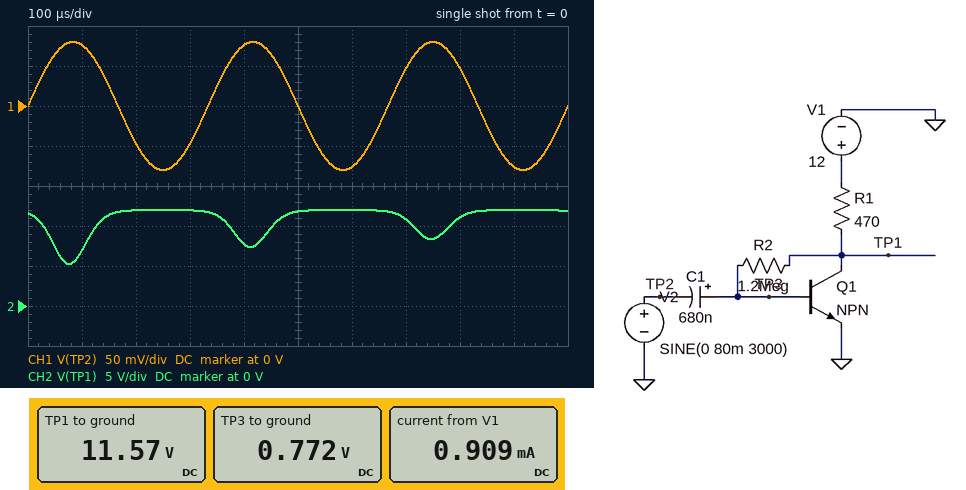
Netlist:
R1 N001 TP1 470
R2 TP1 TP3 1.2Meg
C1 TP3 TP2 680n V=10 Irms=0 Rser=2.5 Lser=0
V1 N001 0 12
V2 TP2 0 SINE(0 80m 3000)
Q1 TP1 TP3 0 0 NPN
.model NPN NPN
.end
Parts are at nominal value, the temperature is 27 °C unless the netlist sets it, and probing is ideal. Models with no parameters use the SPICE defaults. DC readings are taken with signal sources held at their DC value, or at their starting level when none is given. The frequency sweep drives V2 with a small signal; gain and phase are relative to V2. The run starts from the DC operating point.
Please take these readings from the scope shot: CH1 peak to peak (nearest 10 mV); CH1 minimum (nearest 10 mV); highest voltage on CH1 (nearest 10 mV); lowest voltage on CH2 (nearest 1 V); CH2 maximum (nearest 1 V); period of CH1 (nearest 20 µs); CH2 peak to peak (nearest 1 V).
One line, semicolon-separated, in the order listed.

160 mV; -80 mV; 80 mV; 5 V; 12 V; 340 µs; 7 V
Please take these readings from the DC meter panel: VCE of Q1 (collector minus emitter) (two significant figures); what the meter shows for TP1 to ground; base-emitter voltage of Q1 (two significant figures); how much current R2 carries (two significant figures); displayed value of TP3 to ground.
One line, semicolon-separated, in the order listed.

12 V; 11.57 V; 770 mV; 9.0 µA; 0.772 V
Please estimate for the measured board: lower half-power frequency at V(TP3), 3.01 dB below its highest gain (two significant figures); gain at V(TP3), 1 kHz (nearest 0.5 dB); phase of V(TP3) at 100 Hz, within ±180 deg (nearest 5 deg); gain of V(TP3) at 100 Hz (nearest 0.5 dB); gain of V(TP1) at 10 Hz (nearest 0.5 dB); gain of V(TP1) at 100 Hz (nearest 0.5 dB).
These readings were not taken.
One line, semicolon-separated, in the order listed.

85 Hz; 0 dB; 40 deg; -2.5 dB; 5.5 dB; 22.0 dB
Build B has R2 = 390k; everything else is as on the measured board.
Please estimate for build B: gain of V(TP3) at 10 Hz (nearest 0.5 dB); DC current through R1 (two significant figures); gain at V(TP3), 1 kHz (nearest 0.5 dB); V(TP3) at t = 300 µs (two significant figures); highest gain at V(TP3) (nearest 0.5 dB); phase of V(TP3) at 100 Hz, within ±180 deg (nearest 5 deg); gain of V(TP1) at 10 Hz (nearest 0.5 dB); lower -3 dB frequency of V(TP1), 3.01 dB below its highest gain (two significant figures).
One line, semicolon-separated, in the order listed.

-28.5 dB; 2.6 mA; -0.5 dB; 730 mV; 0 dB; 70 deg; 5.0 dB; 260 Hz
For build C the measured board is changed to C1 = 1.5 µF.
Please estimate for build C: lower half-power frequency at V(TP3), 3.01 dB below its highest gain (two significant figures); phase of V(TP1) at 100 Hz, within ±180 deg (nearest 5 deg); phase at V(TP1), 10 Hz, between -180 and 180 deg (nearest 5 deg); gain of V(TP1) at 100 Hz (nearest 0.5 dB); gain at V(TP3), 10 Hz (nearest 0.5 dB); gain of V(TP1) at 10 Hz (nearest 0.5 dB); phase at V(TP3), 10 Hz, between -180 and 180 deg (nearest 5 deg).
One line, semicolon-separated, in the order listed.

38 Hz; -160 deg; -105 deg; 23.5 dB; -12.0 dB; 12.5 dB; 75 deg
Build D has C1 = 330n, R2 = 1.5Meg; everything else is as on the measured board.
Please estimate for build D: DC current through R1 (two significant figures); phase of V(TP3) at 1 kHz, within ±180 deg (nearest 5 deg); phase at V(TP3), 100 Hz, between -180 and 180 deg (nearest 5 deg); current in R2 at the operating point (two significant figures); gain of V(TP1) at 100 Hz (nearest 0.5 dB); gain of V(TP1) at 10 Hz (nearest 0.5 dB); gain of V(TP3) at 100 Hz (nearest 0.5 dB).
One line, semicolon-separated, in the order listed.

730 µA; 10 deg; 55 deg; 7.3 µA; 17.5 dB; -0.5 dB; -4.5 dB
